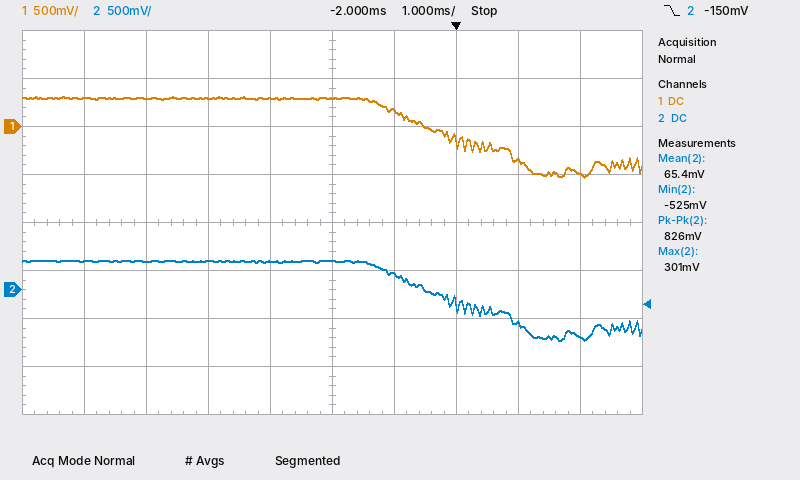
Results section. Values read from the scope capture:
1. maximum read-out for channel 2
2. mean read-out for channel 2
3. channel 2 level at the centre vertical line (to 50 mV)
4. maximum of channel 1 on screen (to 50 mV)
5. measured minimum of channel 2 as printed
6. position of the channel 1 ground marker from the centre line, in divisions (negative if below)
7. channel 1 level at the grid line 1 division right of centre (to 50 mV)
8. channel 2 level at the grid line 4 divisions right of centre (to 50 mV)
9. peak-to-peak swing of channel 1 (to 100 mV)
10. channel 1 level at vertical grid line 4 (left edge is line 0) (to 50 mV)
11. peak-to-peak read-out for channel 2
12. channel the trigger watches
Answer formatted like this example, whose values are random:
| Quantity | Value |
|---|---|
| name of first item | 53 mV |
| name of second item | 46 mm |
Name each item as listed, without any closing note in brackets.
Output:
| Quantity | Value |
|---|---|
| maximum read-out for channel 2 | 301 mV |
| mean read-out for channel 2 | 65.4 mV |
| channel 2 level at the centre vertical line | 300 mV |
| maximum of channel 1 on screen | 300 mV |
| measured minimum of channel 2 as printed | -525 mV |
| position of the channel 1 ground marker from the centre line, in divisions | +2.0 div |
| channel 1 level at the grid line 1 division right of centre | 150 mV |
| channel 2 level at the grid line 4 divisions right of centre | -500 mV |
| peak-to-peak swing of channel 1 | 800 mV |
| channel 1 level at vertical grid line 4 (left edge is line 0) | 300 mV |
| peak-to-peak read-out for channel 2 | 826 mV |
| channel the trigger watches | channel 2 |
